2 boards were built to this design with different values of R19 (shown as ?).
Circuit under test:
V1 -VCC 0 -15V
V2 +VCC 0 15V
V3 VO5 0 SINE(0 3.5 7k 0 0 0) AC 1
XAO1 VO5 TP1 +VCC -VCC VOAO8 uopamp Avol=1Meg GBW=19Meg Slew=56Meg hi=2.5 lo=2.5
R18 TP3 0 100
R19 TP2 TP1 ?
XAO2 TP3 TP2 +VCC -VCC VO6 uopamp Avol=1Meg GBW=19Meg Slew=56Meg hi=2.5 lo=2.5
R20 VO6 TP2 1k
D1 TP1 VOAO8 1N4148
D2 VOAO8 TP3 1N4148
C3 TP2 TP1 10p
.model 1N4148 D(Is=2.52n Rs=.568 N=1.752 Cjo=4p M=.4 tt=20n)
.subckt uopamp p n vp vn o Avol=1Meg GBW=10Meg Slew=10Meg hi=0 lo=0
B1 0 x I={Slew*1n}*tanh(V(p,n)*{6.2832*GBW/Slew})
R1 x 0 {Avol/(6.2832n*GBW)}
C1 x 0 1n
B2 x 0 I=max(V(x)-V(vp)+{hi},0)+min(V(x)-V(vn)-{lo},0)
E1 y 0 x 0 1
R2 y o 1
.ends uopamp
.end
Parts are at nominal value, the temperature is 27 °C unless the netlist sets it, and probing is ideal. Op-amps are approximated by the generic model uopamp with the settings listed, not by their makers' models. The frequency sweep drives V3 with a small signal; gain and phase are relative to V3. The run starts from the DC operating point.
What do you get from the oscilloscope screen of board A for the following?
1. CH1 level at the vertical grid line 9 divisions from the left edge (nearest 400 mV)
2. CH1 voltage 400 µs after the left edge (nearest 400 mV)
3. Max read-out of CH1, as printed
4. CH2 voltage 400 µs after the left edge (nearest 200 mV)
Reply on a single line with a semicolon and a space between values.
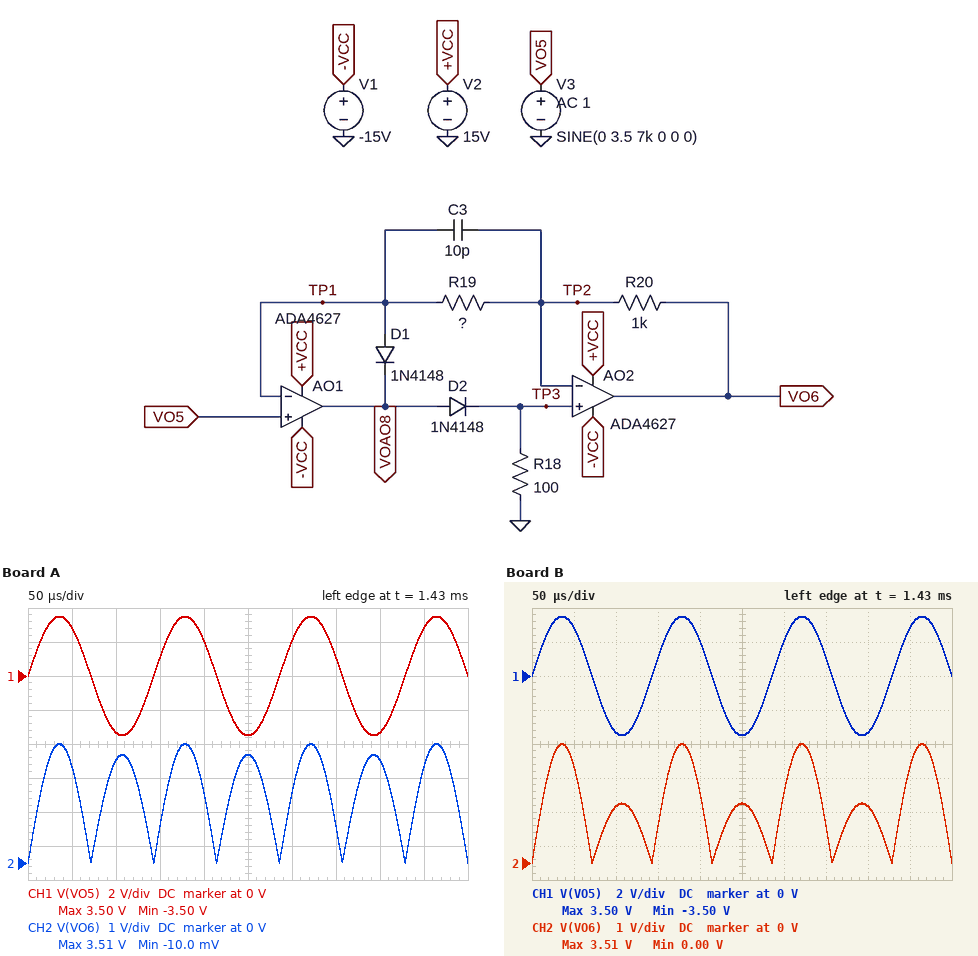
2.8 V; -3.2 V; 3.50 V; 3.0 V
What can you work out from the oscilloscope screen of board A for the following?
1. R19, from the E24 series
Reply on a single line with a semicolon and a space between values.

1.1 kΩ
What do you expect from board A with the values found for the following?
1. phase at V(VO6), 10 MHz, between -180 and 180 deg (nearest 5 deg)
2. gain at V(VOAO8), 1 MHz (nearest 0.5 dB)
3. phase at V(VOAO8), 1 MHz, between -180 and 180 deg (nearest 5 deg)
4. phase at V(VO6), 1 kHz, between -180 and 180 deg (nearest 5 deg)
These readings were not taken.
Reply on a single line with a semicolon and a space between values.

145 deg; 21.5 dB; -90 deg; 155 deg
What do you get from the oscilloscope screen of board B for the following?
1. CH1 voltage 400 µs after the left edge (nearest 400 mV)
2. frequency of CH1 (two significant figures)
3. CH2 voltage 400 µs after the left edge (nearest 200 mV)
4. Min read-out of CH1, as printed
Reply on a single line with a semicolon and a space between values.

-3.2 V; 7.0 kHz; 1.6 V; -3.50 V
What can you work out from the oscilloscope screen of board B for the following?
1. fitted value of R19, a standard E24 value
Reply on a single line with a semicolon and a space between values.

2 kΩ
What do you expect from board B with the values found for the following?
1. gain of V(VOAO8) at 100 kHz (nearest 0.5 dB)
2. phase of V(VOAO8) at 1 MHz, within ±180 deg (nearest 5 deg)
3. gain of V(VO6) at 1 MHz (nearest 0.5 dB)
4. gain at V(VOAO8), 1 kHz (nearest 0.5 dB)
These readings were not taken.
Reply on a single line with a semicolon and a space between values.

39.5 dB; -85 deg; -13.5 dB; 76.0 dB
